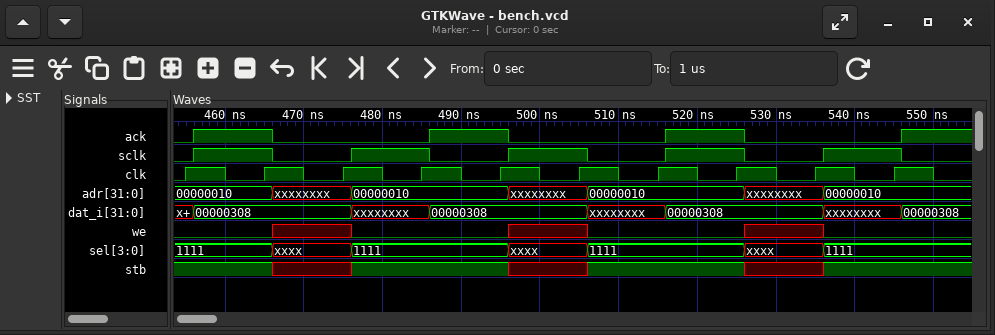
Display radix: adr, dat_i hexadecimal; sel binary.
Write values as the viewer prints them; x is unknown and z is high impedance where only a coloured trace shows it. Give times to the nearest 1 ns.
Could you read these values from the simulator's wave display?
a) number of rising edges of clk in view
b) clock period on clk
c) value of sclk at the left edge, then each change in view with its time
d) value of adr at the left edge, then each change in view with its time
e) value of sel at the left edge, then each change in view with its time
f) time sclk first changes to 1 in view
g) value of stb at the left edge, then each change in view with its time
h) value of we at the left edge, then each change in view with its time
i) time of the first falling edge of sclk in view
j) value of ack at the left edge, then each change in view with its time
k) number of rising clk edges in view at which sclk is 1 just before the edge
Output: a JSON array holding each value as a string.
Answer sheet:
["10", "10 ns", "0, 1 at 456 ns, 0 at 466 ns, 1 at 476 ns, 0 at 486 ns, 1 at 496 ns, 0 at 506 ns, 1 at 516 ns, 0 at 526 ns, 1 at 536 ns, 0 at 546 ns", "00000010, xxxxxxxx at 466 ns, 00000010 at 476 ns, xxxxxxxx at 496 ns, 00000010 at 506 ns, xxxxxxxx at 526 ns, 00000010 at 536 ns", "1111, xxxx at 466 ns, 1111 at 476 ns, xxxx at 496 ns, 1111 at 506 ns, xxxx at 526 ns, 1111 at 536 ns", "456 ns", "1, x at 466 ns, 1 at 476 ns, x at 496 ns, 1 at 506 ns, x at 526 ns, 1 at 536 ns", "0, x at 466 ns, 0 at 476 ns, x at 496 ns, 0 at 506 ns, x at 526 ns, 0 at 536 ns", "466 ns", "0, 1 at 456 ns, 0 at 466 ns, 1 at 486 ns, 0 at 496 ns, 1 at 516 ns, 0 at 526 ns, 1 at 546 ns", "5"]
